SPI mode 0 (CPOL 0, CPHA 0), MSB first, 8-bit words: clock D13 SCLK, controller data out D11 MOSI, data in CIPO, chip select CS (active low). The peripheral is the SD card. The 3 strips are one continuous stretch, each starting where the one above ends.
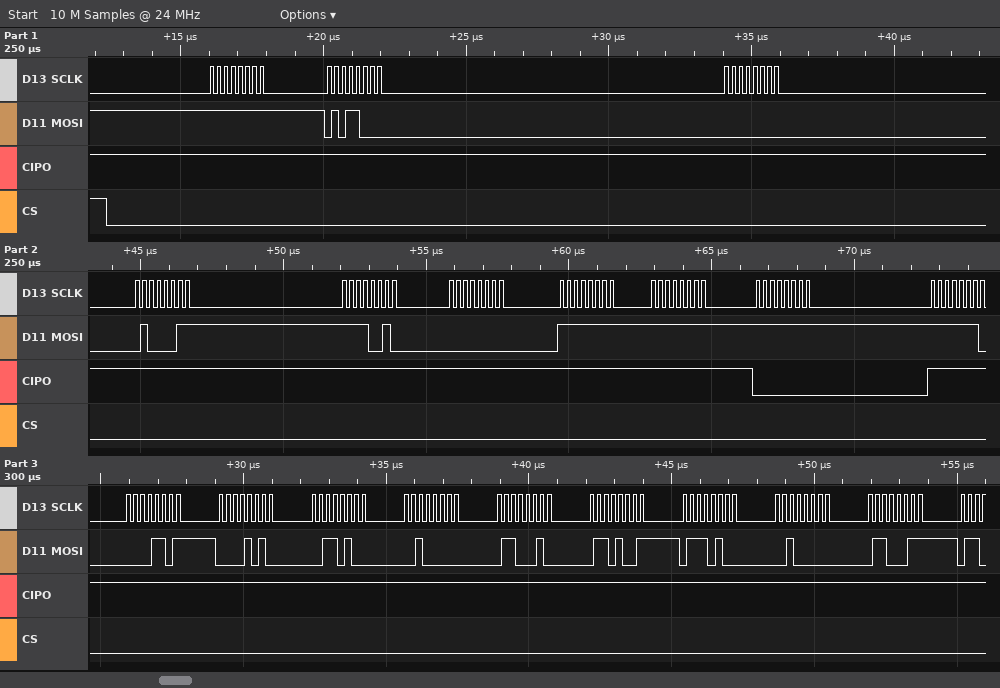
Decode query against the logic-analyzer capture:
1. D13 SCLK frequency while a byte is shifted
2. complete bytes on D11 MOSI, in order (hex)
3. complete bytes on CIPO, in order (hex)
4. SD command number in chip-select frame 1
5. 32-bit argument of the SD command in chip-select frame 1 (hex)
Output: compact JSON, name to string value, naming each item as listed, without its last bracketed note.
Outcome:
{"D13 SCLK frequency while a byte is shifted": "4 MHz", "complete bytes on D11 MOSI, in order": "FF 58 00 43 F2 00 FF FF FF FE 0D 0A 34 20 62 69 74 20 63", "complete bytes on CIPO, in order": "FF FF FF FF FF FF FF FF 00 FF FF FF FF FF FF FF FF FF FF", "SD command number in chip-select frame 1": "CMD24", "32-bit argument of the SD command in chip-select frame 1": "0x0043F200"}
